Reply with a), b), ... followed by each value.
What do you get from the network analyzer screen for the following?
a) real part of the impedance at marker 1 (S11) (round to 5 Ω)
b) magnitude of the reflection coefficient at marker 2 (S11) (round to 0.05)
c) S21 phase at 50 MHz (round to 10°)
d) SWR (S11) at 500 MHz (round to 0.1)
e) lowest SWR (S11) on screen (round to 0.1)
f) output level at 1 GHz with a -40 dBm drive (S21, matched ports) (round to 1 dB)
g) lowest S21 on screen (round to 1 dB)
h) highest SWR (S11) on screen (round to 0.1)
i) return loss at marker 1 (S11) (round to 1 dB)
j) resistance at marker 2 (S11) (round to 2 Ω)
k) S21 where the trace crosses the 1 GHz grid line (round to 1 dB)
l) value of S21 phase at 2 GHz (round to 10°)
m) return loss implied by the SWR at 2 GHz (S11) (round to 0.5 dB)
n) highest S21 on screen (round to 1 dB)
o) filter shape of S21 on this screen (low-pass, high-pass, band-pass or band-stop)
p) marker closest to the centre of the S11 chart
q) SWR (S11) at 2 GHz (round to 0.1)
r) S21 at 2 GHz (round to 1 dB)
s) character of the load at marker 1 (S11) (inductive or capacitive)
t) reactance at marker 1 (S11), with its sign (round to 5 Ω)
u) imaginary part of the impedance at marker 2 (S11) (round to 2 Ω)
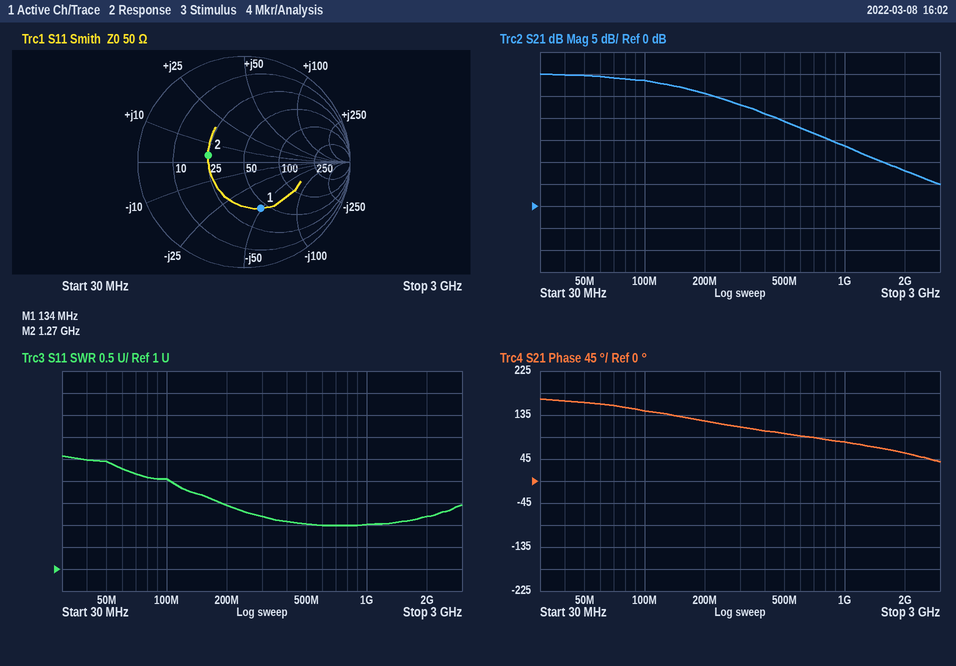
a) 45 Ω
b) 0.35
c) 160°
d) 2.0
e) 2.0
f) -26 dBm
g) 5 dB
h) 3.6
i) 7 dB
j) 24 Ω
k) 14 dB
l) 60°
m) 8.5 dB
n) 30 dB
o) low-pass
p) marker 2
q) 2.2
r) 8 dB
s) capacitive
t) -50 Ω
u) +4 Ω
